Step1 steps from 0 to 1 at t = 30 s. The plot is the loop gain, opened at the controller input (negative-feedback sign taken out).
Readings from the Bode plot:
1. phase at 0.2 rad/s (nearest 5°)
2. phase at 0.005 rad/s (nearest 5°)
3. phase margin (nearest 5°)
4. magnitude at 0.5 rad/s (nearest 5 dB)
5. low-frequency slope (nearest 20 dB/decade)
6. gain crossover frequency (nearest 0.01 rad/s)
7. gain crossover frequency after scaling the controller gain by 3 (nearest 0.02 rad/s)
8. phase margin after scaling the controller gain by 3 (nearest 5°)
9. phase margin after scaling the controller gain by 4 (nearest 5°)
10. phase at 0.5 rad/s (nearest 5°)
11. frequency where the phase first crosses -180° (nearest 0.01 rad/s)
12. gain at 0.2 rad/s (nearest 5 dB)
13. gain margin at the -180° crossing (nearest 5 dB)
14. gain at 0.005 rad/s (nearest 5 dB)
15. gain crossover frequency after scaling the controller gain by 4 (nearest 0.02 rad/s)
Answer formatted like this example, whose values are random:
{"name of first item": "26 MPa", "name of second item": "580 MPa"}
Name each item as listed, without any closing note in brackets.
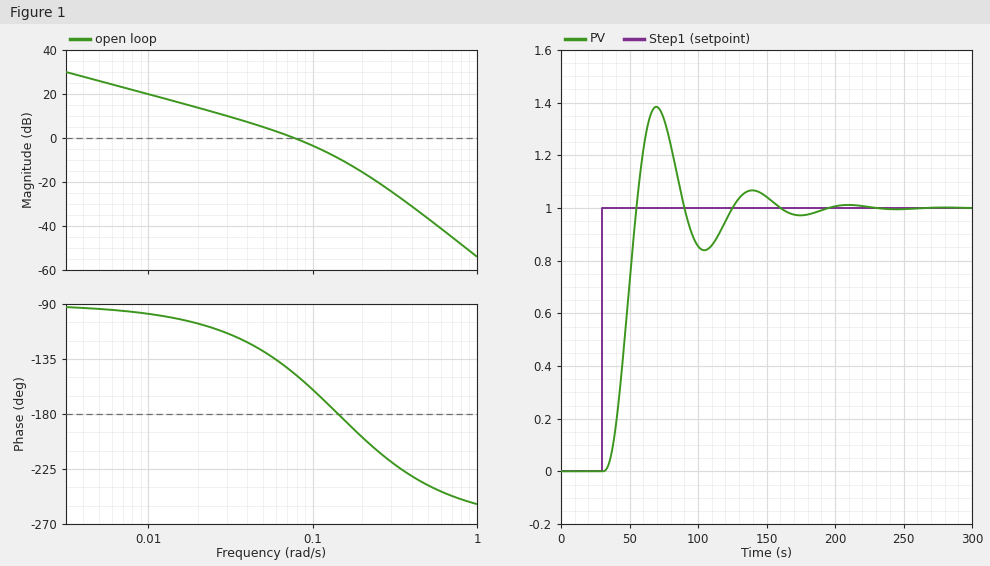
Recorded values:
{"phase at 0.2 rad/s": "-200°", "phase at 0.005 rad/s": "-95°", "phase margin": "35°", "magnitude at 0.5 rad/s": "-35 dB", "low-frequency slope": "-20 dB/decade", "gain crossover frequency": "0.08 rad/s", "gain crossover frequency after scaling the controller gain by 3": "0.14 rad/s", "phase margin after scaling the controller gain by 3": "0°", "phase margin after scaling the controller gain by 4": "-10°", "phase at 0.5 rad/s": "-240°", "frequency where the phase first crosses -180°": "0.14 rad/s", "gain at 0.2 rad/s": "-15 dB", "gain margin at the -180° crossing": "10 dB", "gain at 0.005 rad/s": "25 dB", "gain crossover frequency after scaling the controller gain by 4": "0.16 rad/s"}
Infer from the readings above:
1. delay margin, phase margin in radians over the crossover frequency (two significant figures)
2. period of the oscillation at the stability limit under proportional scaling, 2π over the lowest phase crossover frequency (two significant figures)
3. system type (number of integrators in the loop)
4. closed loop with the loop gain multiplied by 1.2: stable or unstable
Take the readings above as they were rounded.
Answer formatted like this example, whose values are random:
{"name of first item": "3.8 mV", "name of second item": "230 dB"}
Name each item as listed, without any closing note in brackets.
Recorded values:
{"delay margin, phase margin in radians over the crossover frequency": "7.6 s", "period of the oscillation at the stability limit under proportional scaling, 2π over the lowest phase crossover frequency": "45 s", "system type": "1", "closed loop with the loop gain multiplied by 1.2: stable or unstable": "stable"}
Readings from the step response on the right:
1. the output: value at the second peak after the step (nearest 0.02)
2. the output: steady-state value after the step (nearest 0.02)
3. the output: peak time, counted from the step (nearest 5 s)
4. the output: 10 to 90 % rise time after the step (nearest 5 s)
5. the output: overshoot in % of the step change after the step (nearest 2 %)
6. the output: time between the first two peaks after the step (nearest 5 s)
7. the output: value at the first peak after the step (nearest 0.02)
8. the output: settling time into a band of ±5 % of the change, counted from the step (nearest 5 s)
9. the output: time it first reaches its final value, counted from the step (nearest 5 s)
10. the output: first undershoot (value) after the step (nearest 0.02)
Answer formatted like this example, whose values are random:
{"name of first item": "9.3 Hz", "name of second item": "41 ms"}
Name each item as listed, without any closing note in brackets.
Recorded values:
{"the output: value at the second peak after the step": "1.06", "the output: steady-state value after the step": "1.00", "the output: peak time, counted from the step": "40 s", "the output: 10 to 90 % rise time after the step": "15 s", "the output: overshoot in % of the step change after the step": "38 %", "the output: time between the first two peaks after the step": "70 s", "the output: value at the first peak after the step": "1.38", "the output: settling time into a band of ±5 % of the change, counted from the step": "120 s", "the output: time it first reaches its final value, counted from the step": "25 s", "the output: first undershoot (value) after the step": "0.84"}
